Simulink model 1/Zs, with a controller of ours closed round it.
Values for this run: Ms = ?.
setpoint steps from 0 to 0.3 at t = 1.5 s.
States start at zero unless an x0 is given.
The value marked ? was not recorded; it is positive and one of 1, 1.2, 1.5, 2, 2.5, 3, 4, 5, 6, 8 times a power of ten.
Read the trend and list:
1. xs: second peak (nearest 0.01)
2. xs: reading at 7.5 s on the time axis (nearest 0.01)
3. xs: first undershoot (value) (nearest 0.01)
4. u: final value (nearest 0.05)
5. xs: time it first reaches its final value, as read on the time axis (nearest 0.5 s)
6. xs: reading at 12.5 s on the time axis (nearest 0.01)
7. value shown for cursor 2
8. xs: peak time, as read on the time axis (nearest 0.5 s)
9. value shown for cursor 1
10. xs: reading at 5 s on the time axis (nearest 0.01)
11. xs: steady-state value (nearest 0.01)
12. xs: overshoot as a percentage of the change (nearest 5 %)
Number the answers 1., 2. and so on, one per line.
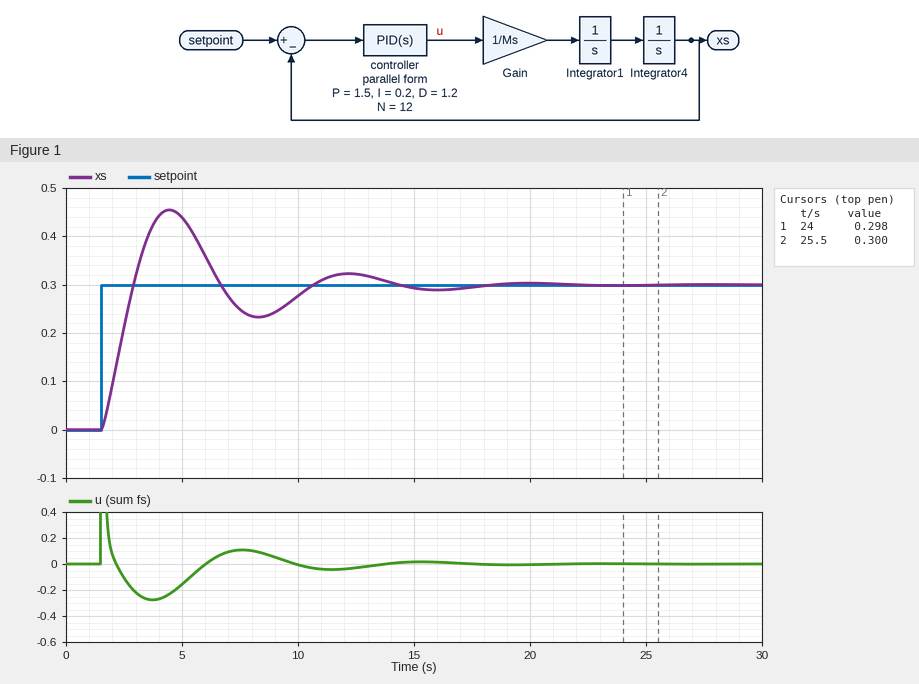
1. 0.32
2. 0.25
3. 0.23
4. 0.00
5. 3.0 s
6. 0.32
7. 0.300
8. 4.5 s
9. 0.298
10. 0.44
11. 0.30
12. 50 %
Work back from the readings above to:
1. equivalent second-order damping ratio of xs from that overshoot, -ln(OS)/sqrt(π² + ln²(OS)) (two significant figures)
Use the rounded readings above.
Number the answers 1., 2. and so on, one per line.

1. 0.22
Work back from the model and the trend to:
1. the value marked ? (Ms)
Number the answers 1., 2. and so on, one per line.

1. 2
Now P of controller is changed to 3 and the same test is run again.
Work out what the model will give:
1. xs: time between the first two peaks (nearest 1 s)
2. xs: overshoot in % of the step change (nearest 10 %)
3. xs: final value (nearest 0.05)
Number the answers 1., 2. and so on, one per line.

1. 5 s
2. 60 %
3. 0.30
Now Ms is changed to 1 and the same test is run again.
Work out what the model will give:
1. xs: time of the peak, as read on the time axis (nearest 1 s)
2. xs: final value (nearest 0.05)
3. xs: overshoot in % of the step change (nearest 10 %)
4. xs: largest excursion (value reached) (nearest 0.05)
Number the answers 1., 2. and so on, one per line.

1. 3 s
2. 0.30
3. 40 %
4. 0.40
